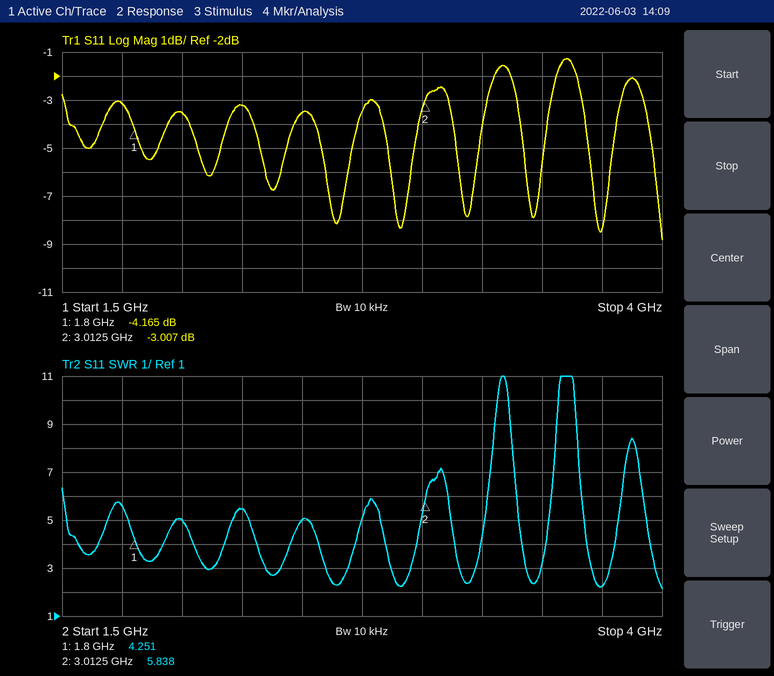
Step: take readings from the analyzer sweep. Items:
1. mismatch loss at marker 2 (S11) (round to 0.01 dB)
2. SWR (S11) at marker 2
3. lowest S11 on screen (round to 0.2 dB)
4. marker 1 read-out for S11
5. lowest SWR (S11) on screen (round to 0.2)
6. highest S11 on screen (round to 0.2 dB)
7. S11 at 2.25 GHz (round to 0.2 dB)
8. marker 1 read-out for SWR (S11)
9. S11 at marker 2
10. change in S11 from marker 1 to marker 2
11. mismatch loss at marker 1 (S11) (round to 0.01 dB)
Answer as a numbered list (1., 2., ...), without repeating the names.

1. 3.01 dB
2. 5.838
3. -8.8 dB
4. -4.165 dB
5. 2.2
6. -1.2 dB
7. -3.2 dB
8. 4.251
9. -3.007 dB
10. 1.158 dB
11. 2.10 dB
